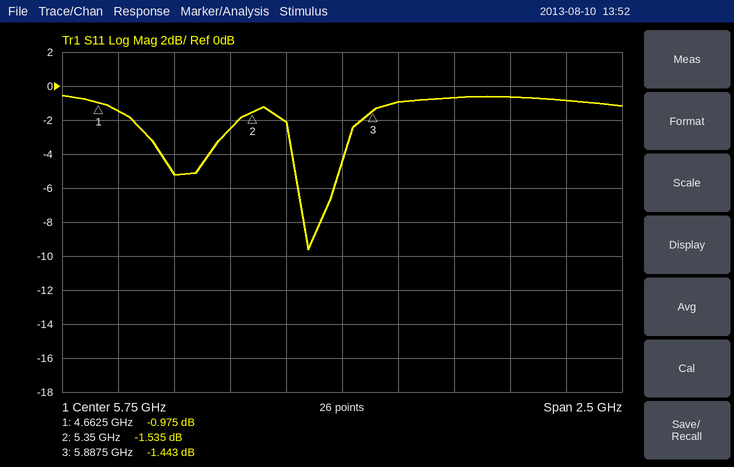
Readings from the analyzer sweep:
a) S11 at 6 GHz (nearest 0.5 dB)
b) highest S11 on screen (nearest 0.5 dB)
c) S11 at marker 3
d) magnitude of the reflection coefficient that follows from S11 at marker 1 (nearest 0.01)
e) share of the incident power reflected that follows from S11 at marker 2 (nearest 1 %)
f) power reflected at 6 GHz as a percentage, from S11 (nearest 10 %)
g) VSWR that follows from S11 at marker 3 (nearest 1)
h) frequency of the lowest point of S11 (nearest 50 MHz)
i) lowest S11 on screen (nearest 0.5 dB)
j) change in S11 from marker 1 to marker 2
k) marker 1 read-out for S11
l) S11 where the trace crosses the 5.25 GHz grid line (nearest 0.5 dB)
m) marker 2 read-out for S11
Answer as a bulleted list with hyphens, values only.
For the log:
- -1.0 dB
- -0.5 dB
- -1.443 dB
- 0.89
- 70 %
- 80 %
- 12
- 5.60 GHz
- -9.5 dB
- -0.560 dB
- -0.975 dB
- -2.5 dB
- -1.535 dB
